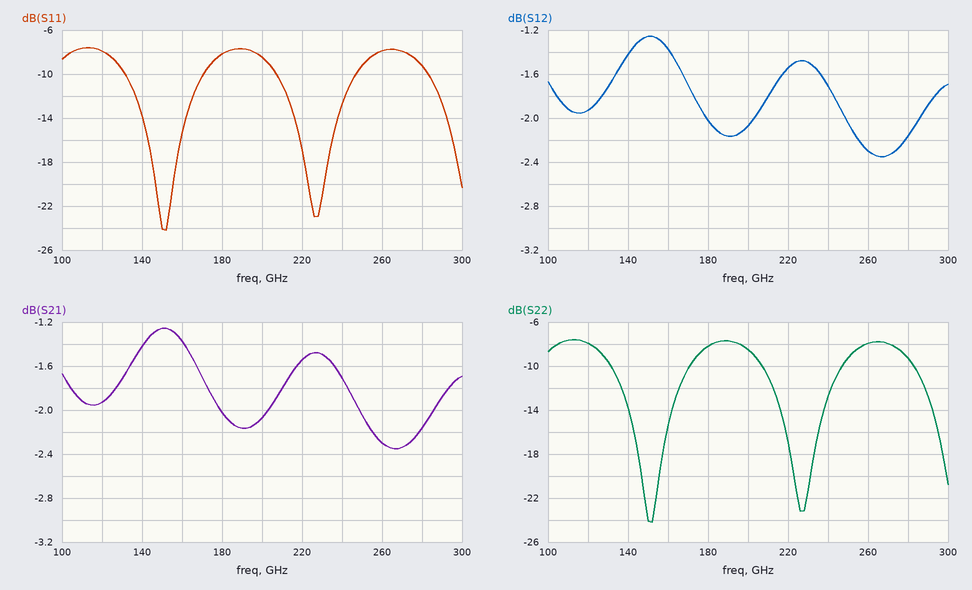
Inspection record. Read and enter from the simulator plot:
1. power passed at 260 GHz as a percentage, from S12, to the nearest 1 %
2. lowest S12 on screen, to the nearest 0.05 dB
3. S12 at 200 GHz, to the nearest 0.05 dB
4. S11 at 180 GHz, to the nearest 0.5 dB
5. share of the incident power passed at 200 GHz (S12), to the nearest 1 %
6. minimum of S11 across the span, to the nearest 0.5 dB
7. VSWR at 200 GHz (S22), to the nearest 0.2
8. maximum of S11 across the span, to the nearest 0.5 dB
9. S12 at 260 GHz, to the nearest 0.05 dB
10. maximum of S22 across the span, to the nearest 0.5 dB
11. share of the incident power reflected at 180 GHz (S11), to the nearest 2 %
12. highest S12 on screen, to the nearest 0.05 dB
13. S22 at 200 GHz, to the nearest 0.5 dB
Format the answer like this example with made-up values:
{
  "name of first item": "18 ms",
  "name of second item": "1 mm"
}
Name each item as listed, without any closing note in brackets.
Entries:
{
  "power passed at 260 GHz as a percentage, from S12, to the nearest 1 %": "59 %",
  "lowest S12 on screen, to the nearest 0.05 dB": "-2.35 dB",
  "S12 at 200 GHz, to the nearest 0.05 dB": "-2.05 dB",
  "S11 at 180 GHz, to the nearest 0.5 dB": "-8.0 dB",
  "share of the incident power passed at 200 GHz (S12), to the nearest 1 %": "62 %",
  "minimum of S11 across the span, to the nearest 0.5 dB": "-24.0 dB",
  "VSWR at 200 GHz (S22), to the nearest 0.2": "2.2",
  "maximum of S11 across the span, to the nearest 0.5 dB": "-7.5 dB",
  "S12 at 260 GHz, to the nearest 0.05 dB": "-2.30 dB",
  "maximum of S22 across the span, to the nearest 0.5 dB": "-7.5 dB",
  "share of the incident power reflected at 180 GHz (S11), to the nearest 2 %": "16 %",
  "highest S12 on screen, to the nearest 0.05 dB": "-1.25 dB",
  "S22 at 200 GHz, to the nearest 0.5 dB": "-8.5 dB"
}
